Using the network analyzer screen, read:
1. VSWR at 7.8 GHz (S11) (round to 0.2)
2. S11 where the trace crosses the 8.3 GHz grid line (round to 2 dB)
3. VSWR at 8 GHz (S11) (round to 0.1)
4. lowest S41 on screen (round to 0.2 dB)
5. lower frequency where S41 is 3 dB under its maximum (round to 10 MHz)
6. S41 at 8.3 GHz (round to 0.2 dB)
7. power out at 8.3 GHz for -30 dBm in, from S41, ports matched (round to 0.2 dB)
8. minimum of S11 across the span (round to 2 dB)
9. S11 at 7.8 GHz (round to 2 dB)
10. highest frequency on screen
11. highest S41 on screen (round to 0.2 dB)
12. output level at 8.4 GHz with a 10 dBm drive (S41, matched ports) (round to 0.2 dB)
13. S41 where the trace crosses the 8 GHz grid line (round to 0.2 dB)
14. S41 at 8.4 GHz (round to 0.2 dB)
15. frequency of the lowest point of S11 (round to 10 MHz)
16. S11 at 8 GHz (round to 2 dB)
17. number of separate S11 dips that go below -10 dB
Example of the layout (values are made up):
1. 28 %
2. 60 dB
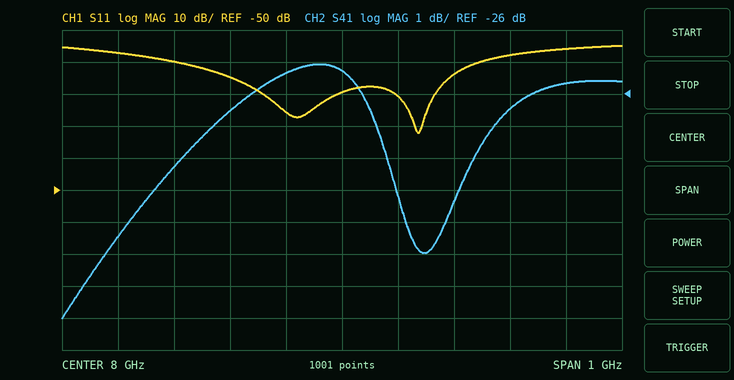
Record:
1. 1.4
2. -8 dB
3. 1.2
4. -33.0 dB
5. 7.71 GHz
6. -26.4 dB
7. -56.4 dBm
8. -32 dB
9. -14 dB
10. 8.5 GHz
11. -25.0 dB
12. -15.6 dBm
13. -25.2 dB
14. -25.6 dB
15. 8.14 GHz
16. -20 dB
17. 2
